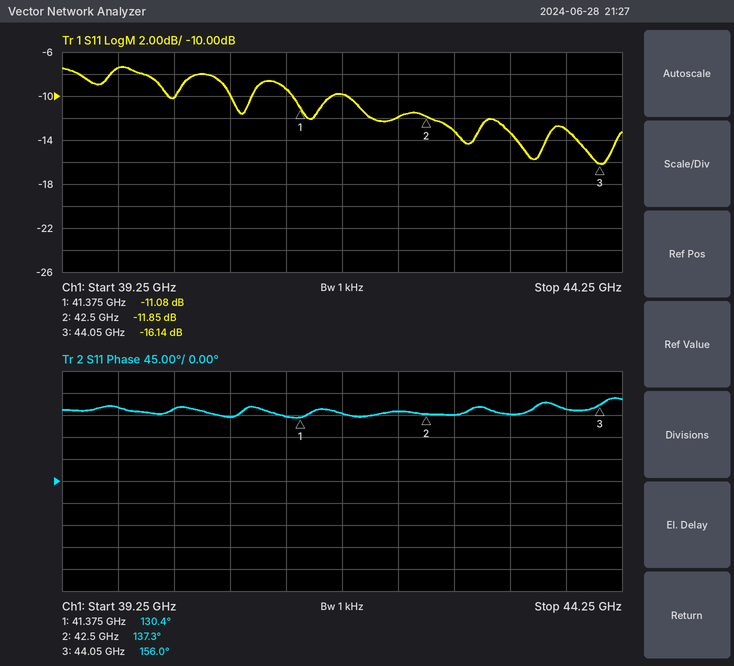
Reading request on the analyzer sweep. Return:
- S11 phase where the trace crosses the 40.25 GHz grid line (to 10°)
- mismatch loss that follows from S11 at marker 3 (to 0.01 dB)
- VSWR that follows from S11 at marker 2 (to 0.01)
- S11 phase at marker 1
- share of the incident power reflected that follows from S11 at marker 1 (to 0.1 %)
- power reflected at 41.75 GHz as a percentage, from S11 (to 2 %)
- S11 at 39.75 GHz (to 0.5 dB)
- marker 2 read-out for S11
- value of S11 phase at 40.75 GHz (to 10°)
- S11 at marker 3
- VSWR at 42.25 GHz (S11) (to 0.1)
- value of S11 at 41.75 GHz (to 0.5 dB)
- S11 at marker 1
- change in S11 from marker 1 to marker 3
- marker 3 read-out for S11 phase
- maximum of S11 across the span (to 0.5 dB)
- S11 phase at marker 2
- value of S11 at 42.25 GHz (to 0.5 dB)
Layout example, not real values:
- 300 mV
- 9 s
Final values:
- 150°
- 0.11 dB
- 1.69
- 130.4°
- 7.8 %
- 10 %
- -7.5 dB
- -11.85 dB
- 130°
- -16.14 dB
- 1.7
- -10.0 dB
- -11.08 dB
- -5.06 dB
- 156.0°
- -7.5 dB
- 137.3°
- -12.0 dB
